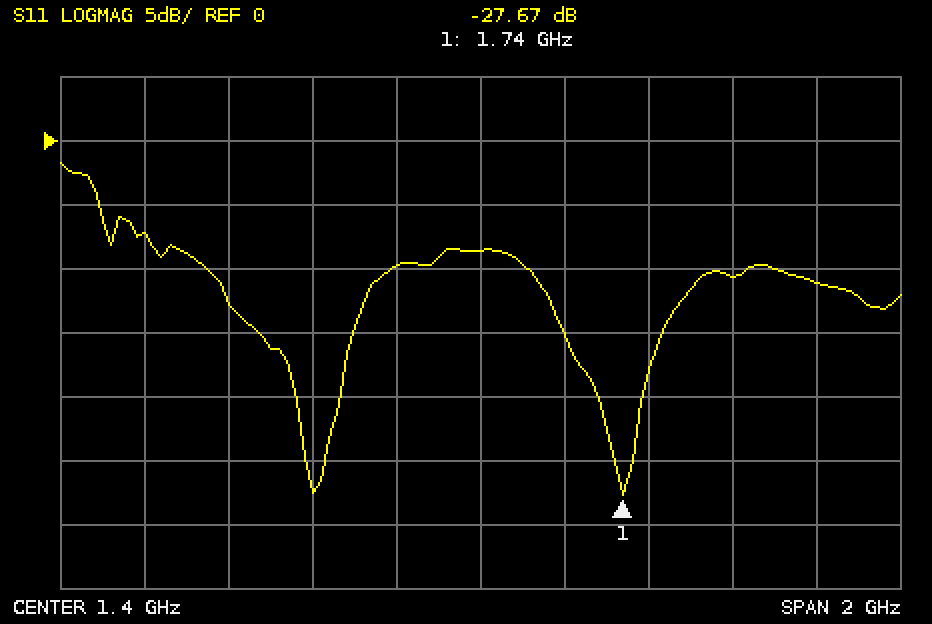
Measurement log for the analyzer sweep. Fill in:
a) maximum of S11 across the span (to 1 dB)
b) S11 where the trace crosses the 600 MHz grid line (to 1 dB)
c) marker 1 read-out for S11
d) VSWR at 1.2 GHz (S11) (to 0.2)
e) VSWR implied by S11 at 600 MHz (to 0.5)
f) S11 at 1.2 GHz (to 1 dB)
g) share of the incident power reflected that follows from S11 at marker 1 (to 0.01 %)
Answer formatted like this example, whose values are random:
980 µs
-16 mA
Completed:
-2 dB
-7 dB
-27.67 dB
2.0
2.5
-10 dB
0.17 %
